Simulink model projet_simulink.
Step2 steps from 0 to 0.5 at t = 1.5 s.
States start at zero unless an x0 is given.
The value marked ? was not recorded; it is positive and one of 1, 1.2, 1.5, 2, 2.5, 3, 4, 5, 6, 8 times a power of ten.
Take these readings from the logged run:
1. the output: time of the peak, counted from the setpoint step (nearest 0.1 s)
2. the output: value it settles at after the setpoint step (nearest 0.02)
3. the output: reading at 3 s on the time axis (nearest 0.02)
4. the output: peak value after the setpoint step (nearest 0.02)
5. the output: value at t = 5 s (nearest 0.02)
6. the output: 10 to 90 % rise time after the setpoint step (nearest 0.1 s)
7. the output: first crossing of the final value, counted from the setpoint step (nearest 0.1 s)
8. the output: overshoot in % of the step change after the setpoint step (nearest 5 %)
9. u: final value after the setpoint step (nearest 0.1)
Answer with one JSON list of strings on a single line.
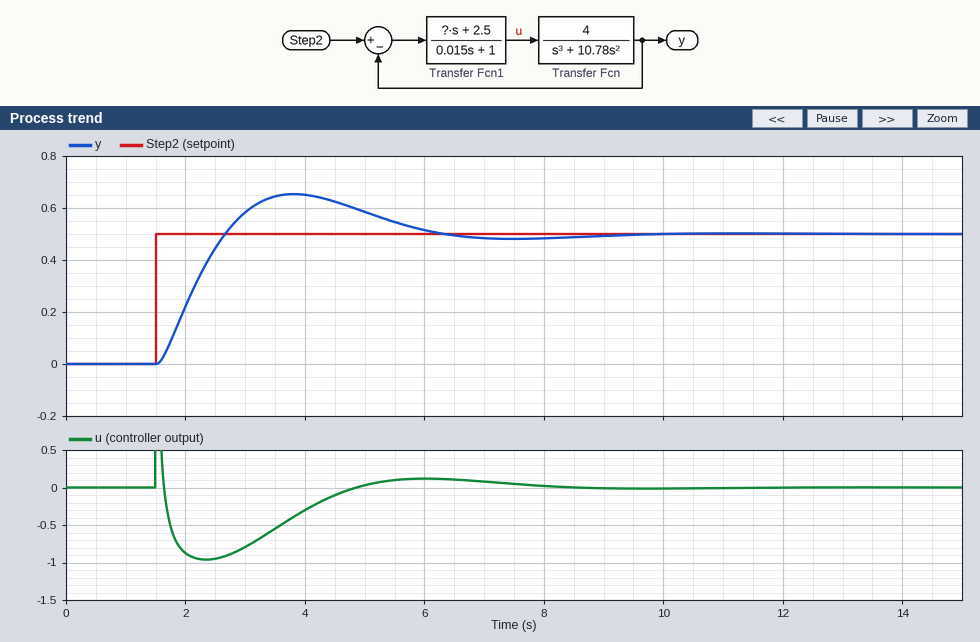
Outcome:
["2.3 s", "0.50", "0.58", "0.66", "0.58", "0.8 s", "1.2 s", "30 %", "0.0"]
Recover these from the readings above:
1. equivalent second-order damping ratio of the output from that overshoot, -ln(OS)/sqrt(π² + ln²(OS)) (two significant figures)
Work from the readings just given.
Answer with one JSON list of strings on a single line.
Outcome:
["0.36"]
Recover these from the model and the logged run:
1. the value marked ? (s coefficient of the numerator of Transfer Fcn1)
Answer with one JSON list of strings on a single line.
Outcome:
["3"]
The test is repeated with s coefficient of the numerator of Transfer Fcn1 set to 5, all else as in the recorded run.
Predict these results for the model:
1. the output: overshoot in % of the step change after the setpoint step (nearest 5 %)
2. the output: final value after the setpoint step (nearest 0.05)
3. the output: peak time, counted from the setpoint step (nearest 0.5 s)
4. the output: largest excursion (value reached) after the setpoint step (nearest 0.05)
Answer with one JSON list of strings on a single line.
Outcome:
["15 %", "0.50", "2.0 s", "0.60"]
